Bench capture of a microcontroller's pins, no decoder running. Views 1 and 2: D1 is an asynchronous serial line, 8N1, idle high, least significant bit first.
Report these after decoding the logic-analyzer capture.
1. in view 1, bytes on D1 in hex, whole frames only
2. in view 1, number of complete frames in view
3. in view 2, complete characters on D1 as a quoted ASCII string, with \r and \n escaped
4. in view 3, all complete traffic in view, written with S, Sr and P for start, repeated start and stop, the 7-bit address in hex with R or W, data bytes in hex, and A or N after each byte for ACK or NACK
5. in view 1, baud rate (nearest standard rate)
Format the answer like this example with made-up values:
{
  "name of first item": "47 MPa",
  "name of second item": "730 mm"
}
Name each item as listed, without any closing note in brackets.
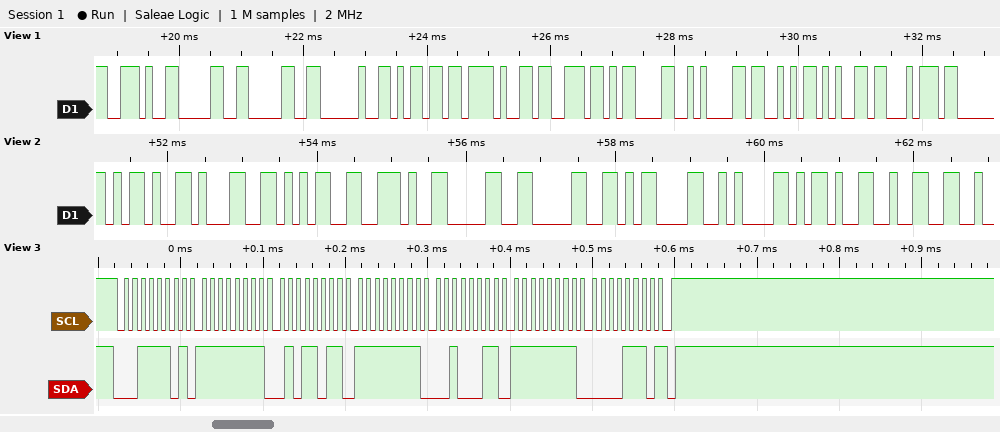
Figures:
{
  "in view 1, bytes on D1 in hex, whole frames only": "2E 30 30 20 6D 2F 73 0D 0A 53 65 74",
  "in view 1, number of complete frames in view": "12",
  "in view 2, complete characters on D1 as a quoted ASCII string, with \\r and \\n escaped": "\"-15.00\\r\\n-2\"",
  "in view 3, all complete traffic in view, written with S, Sr and P for start, repeated start and stop, the 7-bit address in hex with R or W, data bytes in hex, and A or N after each byte for ACK or NACK": "S 1ER A FF A 5B A FF A 23 A FF A 0E N P",
  "in view 1, baud rate": "9600 baud"
}
